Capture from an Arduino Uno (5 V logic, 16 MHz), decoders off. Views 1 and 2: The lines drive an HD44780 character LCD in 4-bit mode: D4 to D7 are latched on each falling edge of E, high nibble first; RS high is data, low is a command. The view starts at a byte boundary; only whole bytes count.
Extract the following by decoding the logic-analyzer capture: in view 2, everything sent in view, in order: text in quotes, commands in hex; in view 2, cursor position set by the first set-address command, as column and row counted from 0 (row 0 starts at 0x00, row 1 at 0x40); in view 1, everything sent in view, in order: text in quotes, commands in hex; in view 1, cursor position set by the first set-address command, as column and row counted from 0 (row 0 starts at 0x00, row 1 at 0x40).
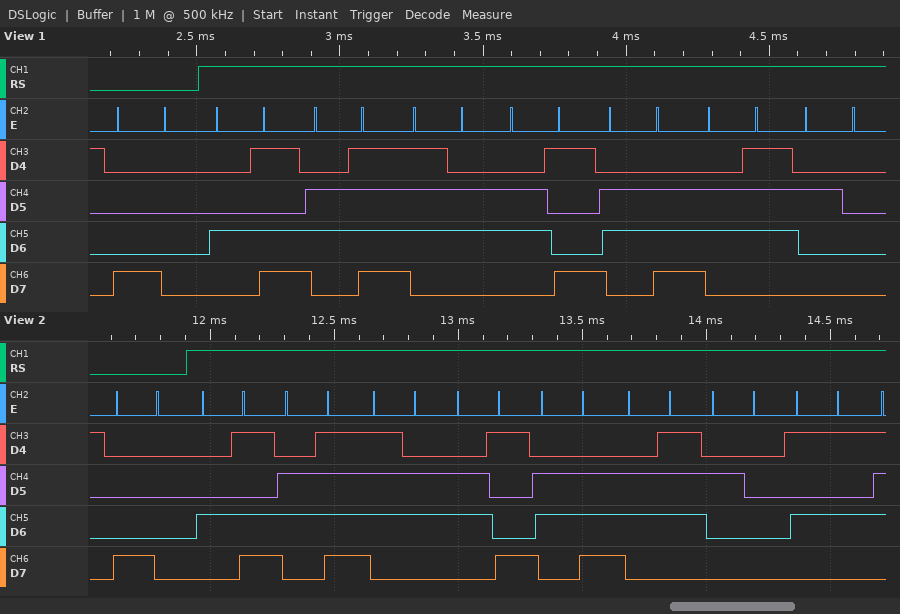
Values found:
0x80 "Moving U"
column 0, row 0
0x80 "Moving "
column 0, row 0
